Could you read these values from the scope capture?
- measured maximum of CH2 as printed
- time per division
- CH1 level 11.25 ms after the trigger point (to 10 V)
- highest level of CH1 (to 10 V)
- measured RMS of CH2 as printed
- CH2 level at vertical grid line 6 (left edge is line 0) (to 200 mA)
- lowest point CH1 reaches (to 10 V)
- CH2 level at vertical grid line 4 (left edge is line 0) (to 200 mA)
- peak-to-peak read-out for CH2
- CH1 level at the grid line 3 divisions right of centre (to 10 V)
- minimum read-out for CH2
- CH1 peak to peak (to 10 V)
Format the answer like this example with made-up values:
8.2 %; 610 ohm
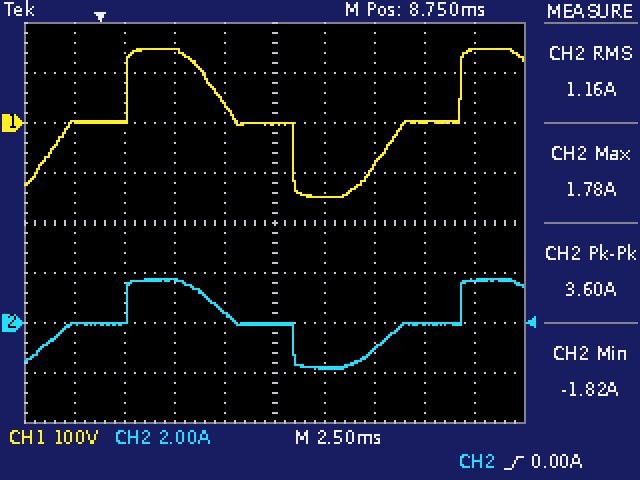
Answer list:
1.78 A; 2.5 ms; -150 V; 150 V; 1.16 A; -1.8 A; -150 V; 400 mA; 3.60 A; 0 V; -1.82 A; 300 V
